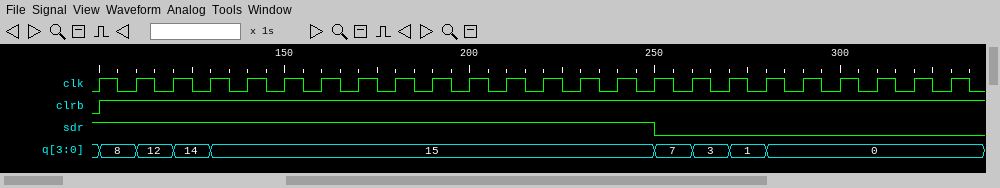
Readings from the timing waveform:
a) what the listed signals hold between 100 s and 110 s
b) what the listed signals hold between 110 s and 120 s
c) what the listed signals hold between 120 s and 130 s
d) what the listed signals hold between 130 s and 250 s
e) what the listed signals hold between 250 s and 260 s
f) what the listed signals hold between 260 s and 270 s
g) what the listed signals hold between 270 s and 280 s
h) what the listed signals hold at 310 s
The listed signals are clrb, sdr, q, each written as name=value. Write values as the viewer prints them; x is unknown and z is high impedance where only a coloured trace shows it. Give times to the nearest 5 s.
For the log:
clrb=1, sdr=1, q=8
clrb=1, sdr=1, q=12
clrb=1, sdr=1, q=14
clrb=1, sdr=1, q=15
clrb=1, sdr=0, q=7
clrb=1, sdr=0, q=3
clrb=1, sdr=0, q=1
clrb=1, sdr=0, q=0
